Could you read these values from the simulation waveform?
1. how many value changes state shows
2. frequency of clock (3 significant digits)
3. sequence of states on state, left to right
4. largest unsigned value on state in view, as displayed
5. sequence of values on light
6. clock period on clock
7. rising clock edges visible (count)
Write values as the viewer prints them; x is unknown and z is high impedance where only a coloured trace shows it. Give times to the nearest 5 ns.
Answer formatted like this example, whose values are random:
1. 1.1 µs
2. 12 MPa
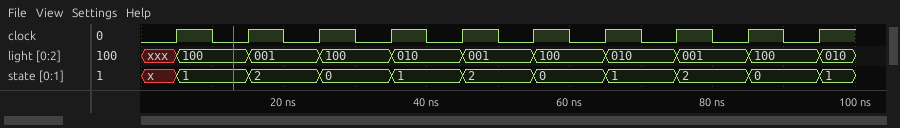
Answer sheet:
1. 10
2. 100 MHz
3. x, 1, 2, 0, 1, 2, 0, 1, 2, 0, 1
4. 2
5. xxx, 100, 001, 100, 010, 001, 100, 010, 001, 100, 010
6. 10 ns
7. 10
